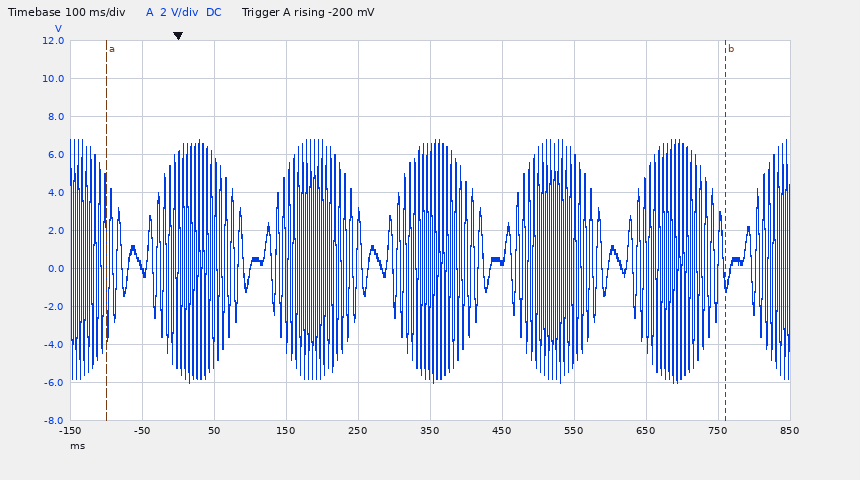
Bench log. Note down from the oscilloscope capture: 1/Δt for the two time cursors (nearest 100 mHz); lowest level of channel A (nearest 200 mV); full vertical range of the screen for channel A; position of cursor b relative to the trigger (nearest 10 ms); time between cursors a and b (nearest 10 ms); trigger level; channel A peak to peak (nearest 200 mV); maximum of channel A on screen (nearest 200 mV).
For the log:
1.2 Hz
-6.0 V
20 V
+760 ms
860 ms
-200 mV
12.8 V
6.8 V
